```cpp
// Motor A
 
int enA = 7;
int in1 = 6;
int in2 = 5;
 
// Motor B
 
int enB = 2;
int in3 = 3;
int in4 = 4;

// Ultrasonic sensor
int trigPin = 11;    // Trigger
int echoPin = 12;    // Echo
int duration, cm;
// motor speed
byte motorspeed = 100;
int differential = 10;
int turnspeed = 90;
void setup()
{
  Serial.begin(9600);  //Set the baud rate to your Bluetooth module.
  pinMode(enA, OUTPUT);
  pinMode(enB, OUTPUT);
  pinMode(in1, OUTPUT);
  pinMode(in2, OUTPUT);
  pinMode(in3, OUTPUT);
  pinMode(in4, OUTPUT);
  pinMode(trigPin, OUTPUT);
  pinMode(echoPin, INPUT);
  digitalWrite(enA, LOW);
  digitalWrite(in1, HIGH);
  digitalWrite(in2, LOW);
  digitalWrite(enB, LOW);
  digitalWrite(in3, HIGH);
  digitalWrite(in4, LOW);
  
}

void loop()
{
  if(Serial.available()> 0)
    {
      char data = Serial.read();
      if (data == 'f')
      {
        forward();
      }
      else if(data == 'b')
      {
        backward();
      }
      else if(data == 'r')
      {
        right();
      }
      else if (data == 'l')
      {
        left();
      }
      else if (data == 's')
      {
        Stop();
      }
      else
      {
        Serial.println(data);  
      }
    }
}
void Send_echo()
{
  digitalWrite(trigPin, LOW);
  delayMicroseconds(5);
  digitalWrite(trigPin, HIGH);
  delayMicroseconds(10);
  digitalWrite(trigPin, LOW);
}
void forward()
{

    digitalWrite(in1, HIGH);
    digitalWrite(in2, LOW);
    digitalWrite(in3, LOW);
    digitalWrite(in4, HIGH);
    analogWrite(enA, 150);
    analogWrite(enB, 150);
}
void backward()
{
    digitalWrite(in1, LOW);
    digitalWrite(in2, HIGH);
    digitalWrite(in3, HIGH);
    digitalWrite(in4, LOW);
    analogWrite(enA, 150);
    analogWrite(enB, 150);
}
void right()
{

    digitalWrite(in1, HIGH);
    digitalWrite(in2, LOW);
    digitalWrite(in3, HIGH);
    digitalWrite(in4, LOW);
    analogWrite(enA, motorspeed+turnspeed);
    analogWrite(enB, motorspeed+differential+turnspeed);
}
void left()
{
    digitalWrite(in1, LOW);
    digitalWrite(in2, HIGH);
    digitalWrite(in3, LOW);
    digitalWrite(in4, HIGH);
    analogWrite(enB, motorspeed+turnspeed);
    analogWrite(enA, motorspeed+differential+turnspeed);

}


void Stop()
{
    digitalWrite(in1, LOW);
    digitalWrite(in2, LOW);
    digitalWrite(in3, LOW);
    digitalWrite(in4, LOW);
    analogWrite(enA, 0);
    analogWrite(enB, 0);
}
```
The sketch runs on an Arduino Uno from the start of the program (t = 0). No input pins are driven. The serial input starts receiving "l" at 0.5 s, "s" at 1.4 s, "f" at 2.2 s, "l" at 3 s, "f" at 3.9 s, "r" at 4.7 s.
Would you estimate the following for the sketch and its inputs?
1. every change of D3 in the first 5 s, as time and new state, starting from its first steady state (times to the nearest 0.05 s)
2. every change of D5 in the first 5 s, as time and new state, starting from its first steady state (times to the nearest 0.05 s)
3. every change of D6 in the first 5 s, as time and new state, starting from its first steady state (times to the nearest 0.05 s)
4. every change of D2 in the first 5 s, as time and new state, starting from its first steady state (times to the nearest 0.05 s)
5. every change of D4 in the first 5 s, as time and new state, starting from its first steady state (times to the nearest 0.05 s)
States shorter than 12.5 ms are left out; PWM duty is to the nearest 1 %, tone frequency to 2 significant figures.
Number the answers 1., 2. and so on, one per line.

1. 0 s high; 0.5 s low; 4.7 s high
2. 0 s low; 0.5 s high; 1.4 s low; 3 s high; 3.9 s low
3. 0 s high; 0.5 s low; 2.2 s high; 3 s low; 3.9 s high
4. 0 s low; 0.5 s high; 1.4 s low; 2.2 s high
5. 0 s low; 0.5 s high; 1.4 s low; 2.2 s high; 4.7 s low
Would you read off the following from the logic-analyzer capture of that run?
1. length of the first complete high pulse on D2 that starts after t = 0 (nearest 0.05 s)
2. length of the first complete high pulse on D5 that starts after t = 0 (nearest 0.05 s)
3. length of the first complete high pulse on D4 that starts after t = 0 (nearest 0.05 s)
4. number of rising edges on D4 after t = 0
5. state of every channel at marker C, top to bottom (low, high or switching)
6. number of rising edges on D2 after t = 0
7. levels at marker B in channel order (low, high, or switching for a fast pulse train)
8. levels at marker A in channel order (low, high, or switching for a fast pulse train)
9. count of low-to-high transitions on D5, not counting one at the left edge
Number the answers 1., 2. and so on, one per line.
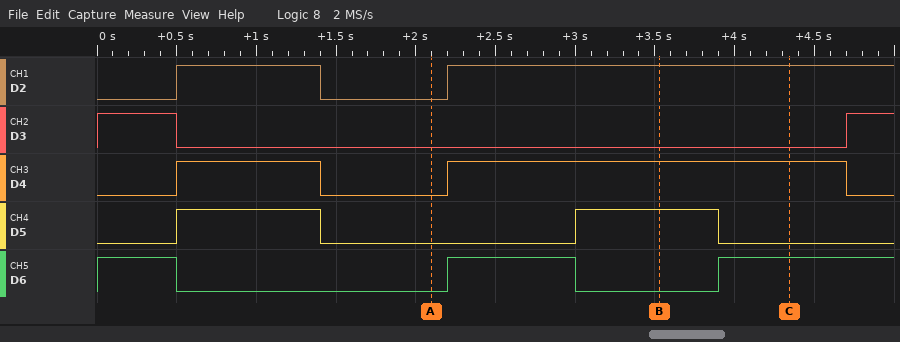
1. 0.90 s
2. 0.90 s
3. 0.90 s
4. 2
5. D2 high, D3 low, D4 high, D5 low, D6 high
6. 2
7. D2 high, D3 low, D4 high, D5 high, D6 low
8. D2 low, D3 low, D4 low, D5 low, D6 low
9. 2
